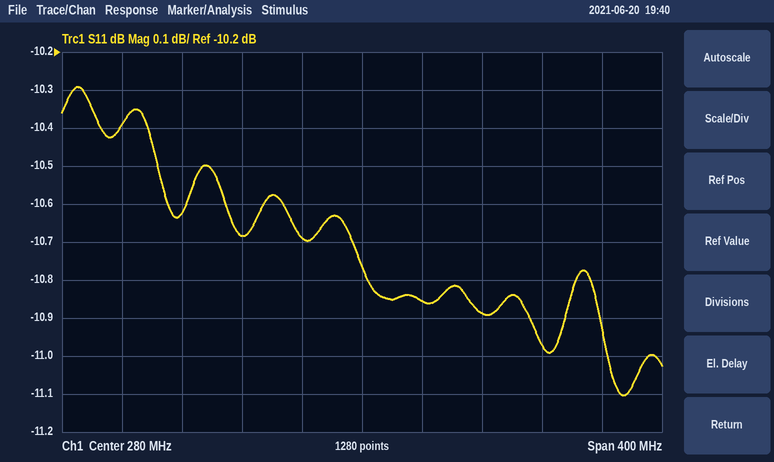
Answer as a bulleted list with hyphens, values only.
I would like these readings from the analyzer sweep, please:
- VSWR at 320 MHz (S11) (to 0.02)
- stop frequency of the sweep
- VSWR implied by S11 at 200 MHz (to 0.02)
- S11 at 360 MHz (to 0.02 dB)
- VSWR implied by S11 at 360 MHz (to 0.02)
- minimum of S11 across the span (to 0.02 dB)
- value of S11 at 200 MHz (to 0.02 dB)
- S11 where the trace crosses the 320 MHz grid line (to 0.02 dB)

- 1.80
- 480 MHz
- 1.82
- -10.88 dB
- 1.80
- -11.10 dB
- -10.68 dB
- -10.86 dB
